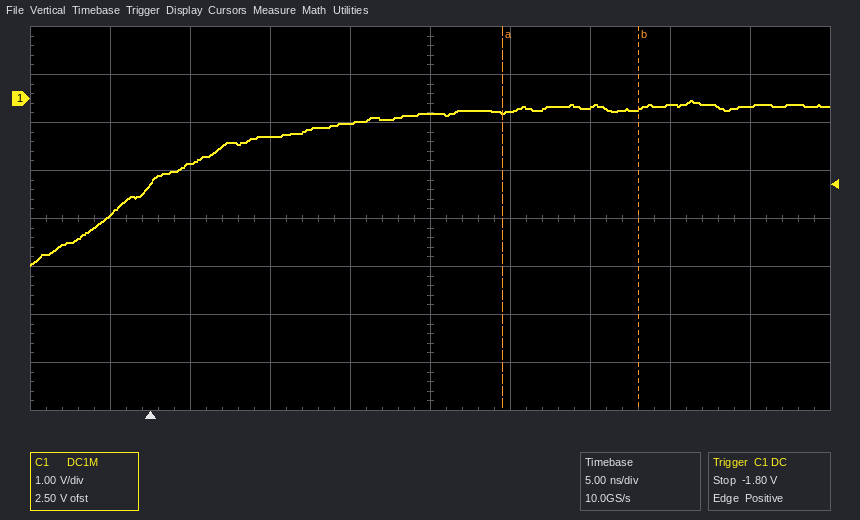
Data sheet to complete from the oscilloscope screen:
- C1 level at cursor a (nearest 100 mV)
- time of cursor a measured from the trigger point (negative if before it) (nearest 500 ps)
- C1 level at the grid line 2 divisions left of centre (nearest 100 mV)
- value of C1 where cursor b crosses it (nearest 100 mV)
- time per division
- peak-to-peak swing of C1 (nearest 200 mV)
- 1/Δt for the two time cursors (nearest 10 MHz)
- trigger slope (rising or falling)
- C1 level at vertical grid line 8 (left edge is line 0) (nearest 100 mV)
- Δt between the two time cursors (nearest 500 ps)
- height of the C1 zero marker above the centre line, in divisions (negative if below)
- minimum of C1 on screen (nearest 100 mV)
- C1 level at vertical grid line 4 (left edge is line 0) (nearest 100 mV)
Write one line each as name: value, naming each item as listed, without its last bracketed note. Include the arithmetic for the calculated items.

C1 level at cursor a: -300 mV
time of cursor a measured from the trigger point (negative if before it): +22.0 ns
C1 level at the grid line 2 divisions left of centre: -800 mV
value of C1 where cursor b crosses it: -200 mV
time per division: 5 ns
peak-to-peak swing of C1: 3.4 V
1/Δt for the two time cursors: 1 / 8.5 ns ≈ 120 MHz
trigger slope: rising
C1 level at vertical grid line 8 (left edge is line 0): -100 mV
Δt between the two time cursors: 8.5 ns
height of the C1 zero marker above the centre line, in divisions: +2.5 div
minimum of C1 on screen: -3.5 V
C1 level at vertical grid line 4 (left edge is line 0): -500 mV
